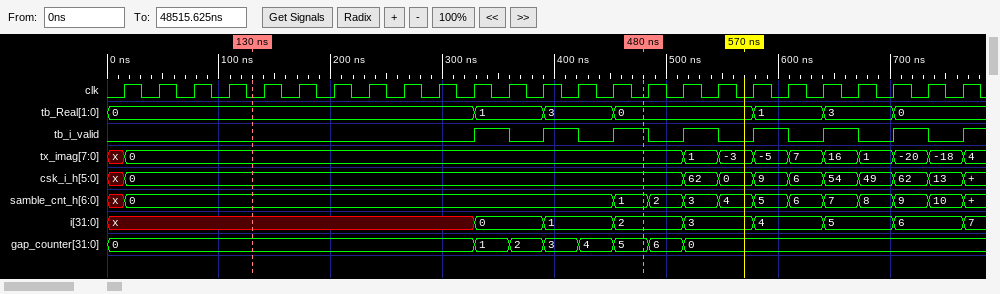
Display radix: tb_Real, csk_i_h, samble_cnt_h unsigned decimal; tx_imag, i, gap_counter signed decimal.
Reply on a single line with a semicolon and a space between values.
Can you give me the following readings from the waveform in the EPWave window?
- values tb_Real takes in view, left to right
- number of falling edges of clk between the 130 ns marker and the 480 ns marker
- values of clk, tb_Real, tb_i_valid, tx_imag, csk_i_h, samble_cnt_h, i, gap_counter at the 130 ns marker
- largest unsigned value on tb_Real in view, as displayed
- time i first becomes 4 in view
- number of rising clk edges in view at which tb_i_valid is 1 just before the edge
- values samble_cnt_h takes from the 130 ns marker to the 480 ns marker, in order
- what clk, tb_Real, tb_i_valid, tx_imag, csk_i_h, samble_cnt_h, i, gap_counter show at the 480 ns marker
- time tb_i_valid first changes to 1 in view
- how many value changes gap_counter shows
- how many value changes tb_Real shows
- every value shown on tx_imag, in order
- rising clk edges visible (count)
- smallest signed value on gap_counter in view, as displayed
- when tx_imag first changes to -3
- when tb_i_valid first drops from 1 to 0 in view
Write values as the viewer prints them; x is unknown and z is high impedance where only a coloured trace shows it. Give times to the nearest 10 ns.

0, 1, 3, 0, 1, 3, 0; 11; clk=0, tb_Real=0, tb_i_valid=0, tx_imag=0, csk_i_h=0, samble_cnt_h=0, i=x, gap_counter=0; 3; 580 ns; 7; 0, 1; clk=0, tb_Real=0, tb_i_valid=1, tx_imag=0, csk_i_h=0, samble_cnt_h=1, i=2, gap_counter=5; 330 ns; 7; 6; x, 0, 1, -3, -5, 7, 16, 1, -20, -18, 4; 25; 0; 550 ns; 360 ns
